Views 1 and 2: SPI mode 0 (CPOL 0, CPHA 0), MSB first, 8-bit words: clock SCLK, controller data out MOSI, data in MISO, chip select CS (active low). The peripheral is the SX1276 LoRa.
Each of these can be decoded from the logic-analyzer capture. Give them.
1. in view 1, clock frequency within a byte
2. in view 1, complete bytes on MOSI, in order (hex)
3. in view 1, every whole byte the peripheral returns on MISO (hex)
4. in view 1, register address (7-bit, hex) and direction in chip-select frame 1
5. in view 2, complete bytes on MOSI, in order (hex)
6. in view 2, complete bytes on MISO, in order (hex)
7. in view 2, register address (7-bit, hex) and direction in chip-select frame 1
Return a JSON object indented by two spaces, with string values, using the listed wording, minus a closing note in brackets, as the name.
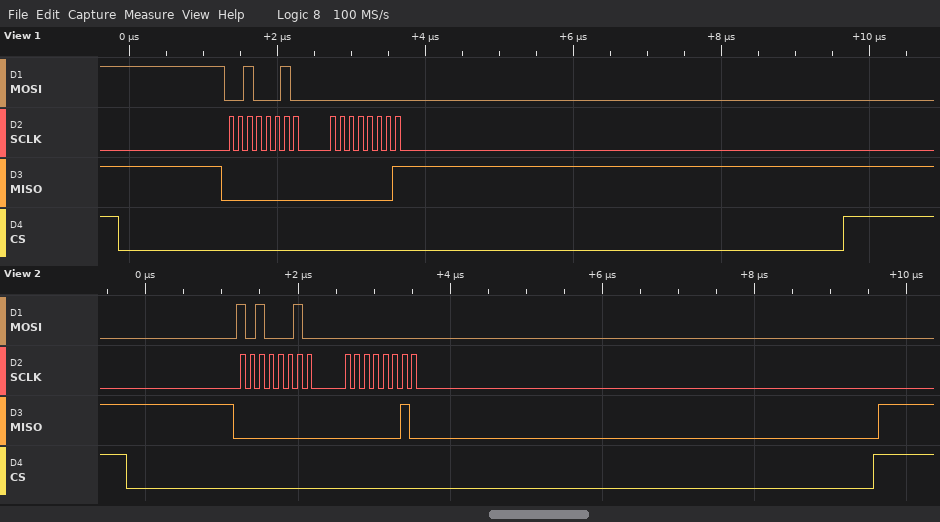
{
  "in view 1, clock frequency within a byte": "8 MHz",
  "in view 1, complete bytes on MOSI, in order": "22 00",
  "in view 1, every whole byte the peripheral returns on MISO": "00 01",
  "in view 1, register address (7-bit, hex) and direction in chip-select frame 1": "0x22 read",
  "in view 2, complete bytes on MOSI, in order": "0xA2 0x00",
  "in view 2, complete bytes on MISO, in order": "0x00 0x02",
  "in view 2, register address (7-bit, hex) and direction in chip-select frame 1": "0x22 write"
}
